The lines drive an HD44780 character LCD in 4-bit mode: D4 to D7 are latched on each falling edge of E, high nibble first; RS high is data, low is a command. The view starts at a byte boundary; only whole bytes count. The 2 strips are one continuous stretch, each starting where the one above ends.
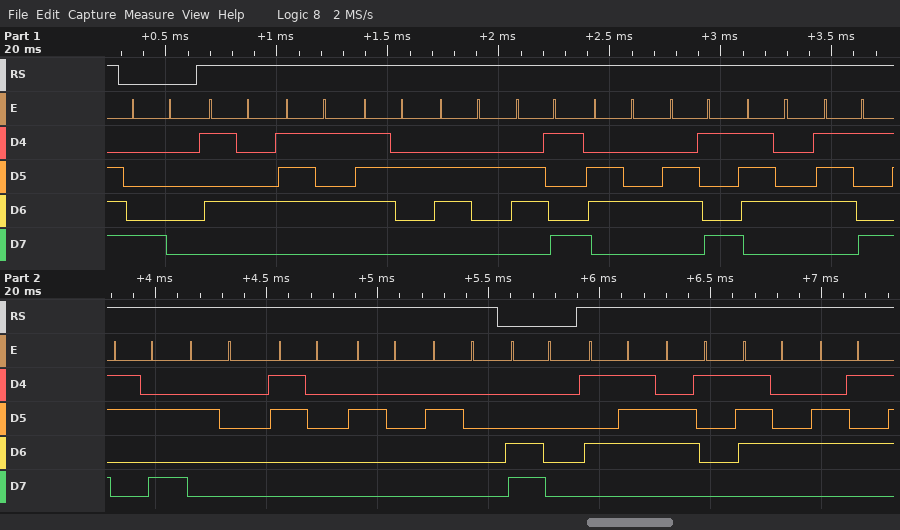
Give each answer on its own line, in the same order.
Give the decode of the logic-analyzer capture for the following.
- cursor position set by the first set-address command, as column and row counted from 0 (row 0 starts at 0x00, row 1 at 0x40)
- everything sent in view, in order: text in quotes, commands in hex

column 0, row 0
0x80 "Turbidity: 0  " 0xC0 "Wate"
